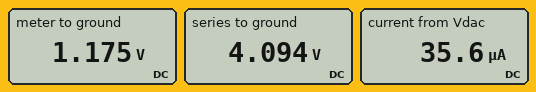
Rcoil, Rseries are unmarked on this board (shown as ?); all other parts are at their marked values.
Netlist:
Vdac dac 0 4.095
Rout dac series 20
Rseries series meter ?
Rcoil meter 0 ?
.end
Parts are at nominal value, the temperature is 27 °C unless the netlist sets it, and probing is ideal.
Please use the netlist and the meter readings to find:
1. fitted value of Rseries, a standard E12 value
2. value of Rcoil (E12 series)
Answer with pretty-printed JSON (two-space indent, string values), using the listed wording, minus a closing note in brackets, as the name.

{
  "fitted value of Rseries, a standard E12 value": "82 kΩ",
  "value of Rcoil": "33 kΩ"
}
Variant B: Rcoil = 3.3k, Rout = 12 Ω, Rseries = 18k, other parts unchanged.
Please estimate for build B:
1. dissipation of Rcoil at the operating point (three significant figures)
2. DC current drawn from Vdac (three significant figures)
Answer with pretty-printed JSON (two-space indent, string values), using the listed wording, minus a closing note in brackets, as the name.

{
  "dissipation of Rcoil at the operating point": "122 µW",
  "DC current drawn from Vdac": "192 µA"
}
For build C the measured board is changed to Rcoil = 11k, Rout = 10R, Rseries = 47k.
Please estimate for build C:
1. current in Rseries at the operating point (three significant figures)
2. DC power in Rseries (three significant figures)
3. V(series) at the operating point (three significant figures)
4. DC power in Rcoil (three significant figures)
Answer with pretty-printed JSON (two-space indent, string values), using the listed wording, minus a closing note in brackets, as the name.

{
  "current in Rseries at the operating point": "70.6 µA",
  "DC power in Rseries": "234 µW",
  "V(series) at the operating point": "4.09 V",
  "DC power in Rcoil": "54.8 µW"
}
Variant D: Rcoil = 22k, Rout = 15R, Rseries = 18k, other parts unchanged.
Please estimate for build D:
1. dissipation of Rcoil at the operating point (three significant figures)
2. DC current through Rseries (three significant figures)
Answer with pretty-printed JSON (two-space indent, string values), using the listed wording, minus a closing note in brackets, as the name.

{
  "dissipation of Rcoil at the operating point": "230 µW",
  "DC current through Rseries": "102 µA"
}
